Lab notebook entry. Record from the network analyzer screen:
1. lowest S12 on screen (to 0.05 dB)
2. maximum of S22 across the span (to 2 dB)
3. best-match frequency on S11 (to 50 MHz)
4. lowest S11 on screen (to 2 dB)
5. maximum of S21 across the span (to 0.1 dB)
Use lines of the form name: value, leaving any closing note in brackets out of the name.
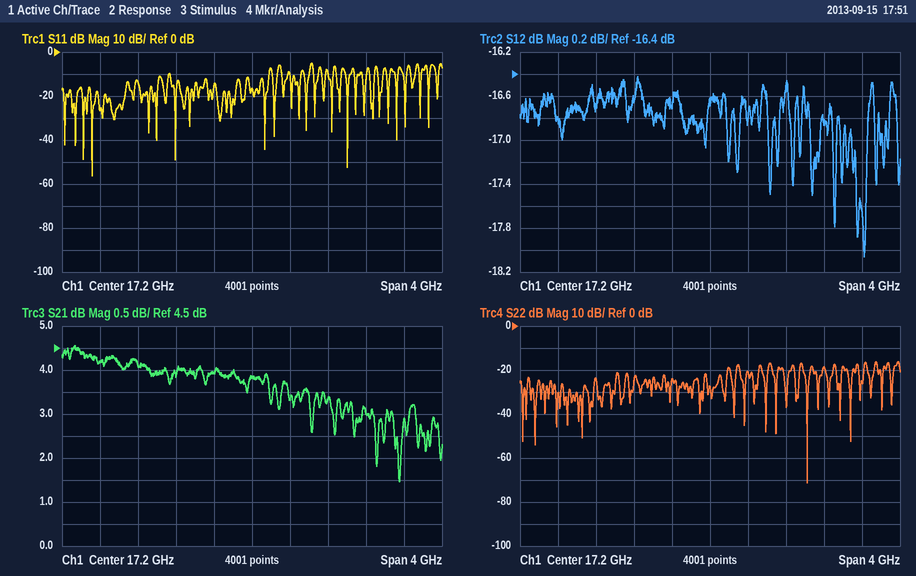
lowest S12 on screen: -18.05 dB
maximum of S22 across the span: -16 dB
best-match frequency on S11: 15.50 GHz
lowest S11 on screen: -56 dB
maximum of S21 across the span: 4.6 dB
